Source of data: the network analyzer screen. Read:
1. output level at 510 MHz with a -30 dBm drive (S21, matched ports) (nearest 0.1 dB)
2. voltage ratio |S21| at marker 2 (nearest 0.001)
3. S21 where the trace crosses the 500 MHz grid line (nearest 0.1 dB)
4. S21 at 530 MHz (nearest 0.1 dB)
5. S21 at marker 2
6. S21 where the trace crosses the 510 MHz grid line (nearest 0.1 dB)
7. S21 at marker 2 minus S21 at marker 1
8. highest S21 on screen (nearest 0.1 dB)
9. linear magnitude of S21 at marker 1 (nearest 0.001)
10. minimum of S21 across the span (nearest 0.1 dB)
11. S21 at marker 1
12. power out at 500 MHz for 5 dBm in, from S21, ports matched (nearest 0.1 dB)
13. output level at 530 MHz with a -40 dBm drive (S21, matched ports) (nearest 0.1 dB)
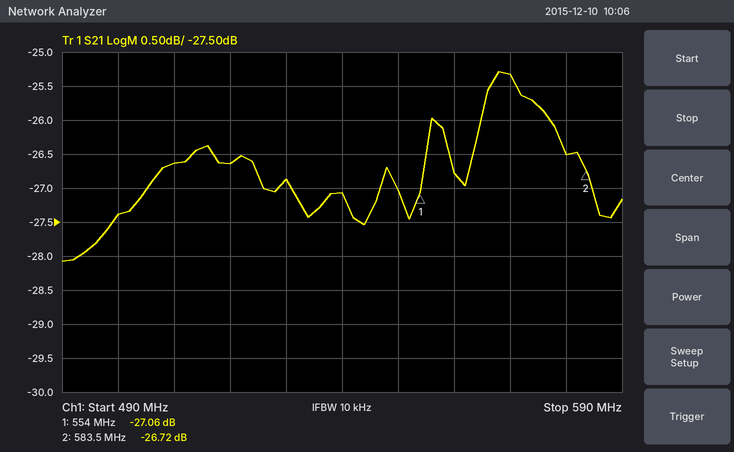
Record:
-56.6 dBm
0.046
-27.4 dB
-26.9 dB
-26.72 dB
-26.6 dB
0.34 dB
-25.3 dB
0.044
-28.1 dB
-27.06 dB
-22.4 dBm
-66.9 dBm
